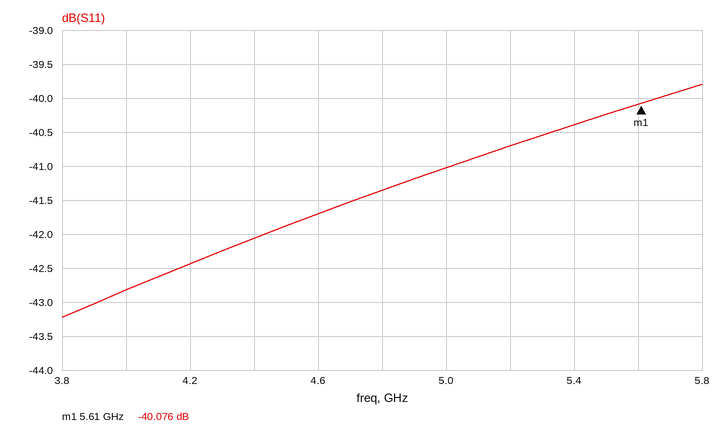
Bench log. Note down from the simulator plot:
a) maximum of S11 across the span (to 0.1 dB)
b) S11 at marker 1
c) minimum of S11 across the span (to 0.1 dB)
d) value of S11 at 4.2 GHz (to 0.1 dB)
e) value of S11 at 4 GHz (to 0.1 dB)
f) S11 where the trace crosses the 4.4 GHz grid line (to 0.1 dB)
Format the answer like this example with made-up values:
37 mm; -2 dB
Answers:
-39.8 dB; -40.076 dB; -43.2 dB; -42.4 dB; -42.8 dB; -42.1 dB
